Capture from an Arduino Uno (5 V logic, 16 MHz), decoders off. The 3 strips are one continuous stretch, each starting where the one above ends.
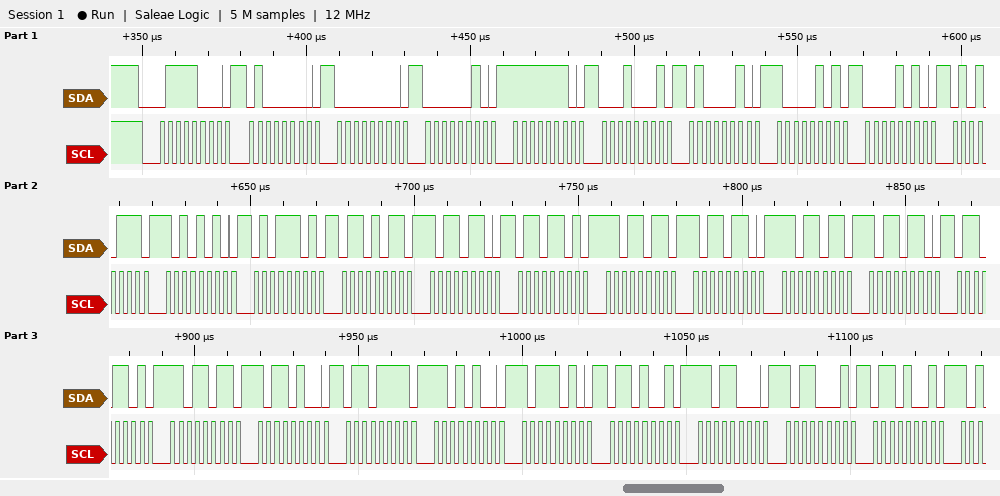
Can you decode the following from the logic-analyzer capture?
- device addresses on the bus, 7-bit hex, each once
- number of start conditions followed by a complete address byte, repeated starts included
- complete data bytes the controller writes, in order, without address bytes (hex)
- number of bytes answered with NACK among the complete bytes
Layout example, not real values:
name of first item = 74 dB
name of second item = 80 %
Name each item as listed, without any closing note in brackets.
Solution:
device addresses on the bus, 7-bit hex, each once = 0x3C
number of start conditions followed by a complete address byte, repeated starts included = 1
complete data bytes the controller writes, in order, without address bytes = 40 00 02 FE 11 42 85 0A 57 AA 5D 6B B6 6D DB B6 DB B6 6D DB B4 6F D4 BA 69 D8 B1 69
number of bytes answered with NACK among the complete bytes = 0
